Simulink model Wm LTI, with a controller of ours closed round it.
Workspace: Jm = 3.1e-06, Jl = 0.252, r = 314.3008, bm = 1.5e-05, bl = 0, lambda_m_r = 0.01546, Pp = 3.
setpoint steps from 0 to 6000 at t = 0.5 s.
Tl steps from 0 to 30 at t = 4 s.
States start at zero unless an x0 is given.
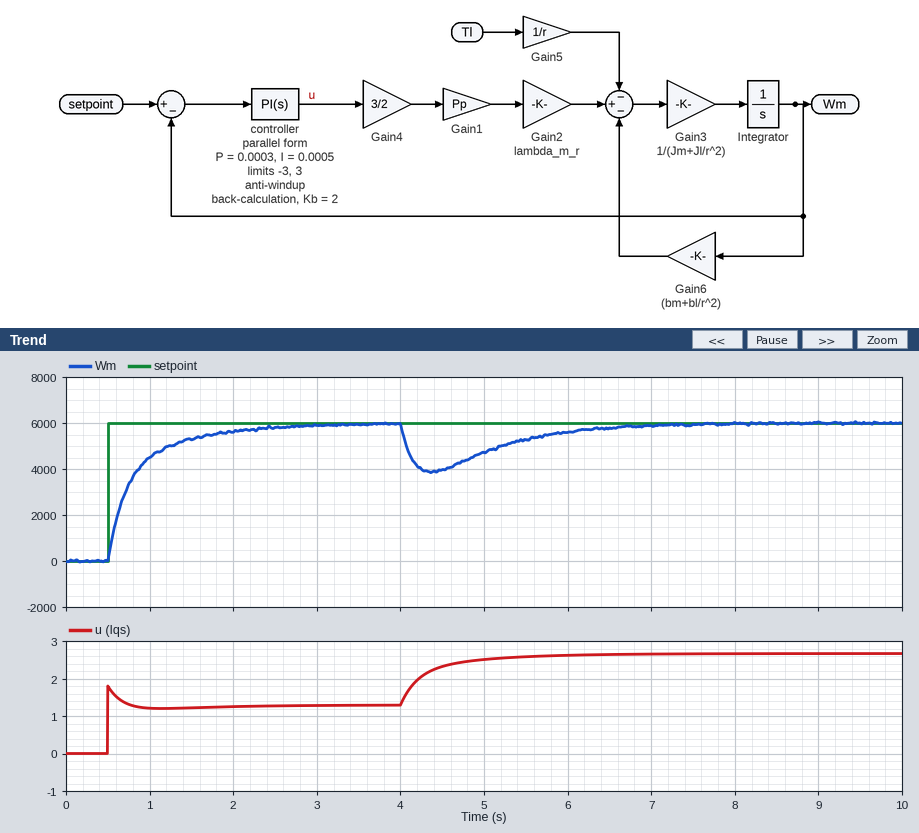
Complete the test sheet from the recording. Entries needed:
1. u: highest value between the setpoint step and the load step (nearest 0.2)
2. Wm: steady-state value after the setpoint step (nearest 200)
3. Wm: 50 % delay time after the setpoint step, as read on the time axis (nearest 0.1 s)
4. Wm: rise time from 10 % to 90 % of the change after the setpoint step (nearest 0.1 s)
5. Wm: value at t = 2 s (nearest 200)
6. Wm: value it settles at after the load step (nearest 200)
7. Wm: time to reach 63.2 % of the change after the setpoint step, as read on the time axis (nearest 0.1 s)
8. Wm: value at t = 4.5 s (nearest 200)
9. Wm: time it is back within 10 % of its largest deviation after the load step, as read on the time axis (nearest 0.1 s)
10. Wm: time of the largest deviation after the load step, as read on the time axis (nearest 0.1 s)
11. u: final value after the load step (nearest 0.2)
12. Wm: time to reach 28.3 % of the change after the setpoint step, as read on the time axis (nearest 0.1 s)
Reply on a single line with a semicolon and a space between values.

1.8; 6000; 0.7 s; 1.1 s; 5600; 6000; 0.8 s; 4000; 6.5 s; 4.4 s; 2.6; 0.6 s
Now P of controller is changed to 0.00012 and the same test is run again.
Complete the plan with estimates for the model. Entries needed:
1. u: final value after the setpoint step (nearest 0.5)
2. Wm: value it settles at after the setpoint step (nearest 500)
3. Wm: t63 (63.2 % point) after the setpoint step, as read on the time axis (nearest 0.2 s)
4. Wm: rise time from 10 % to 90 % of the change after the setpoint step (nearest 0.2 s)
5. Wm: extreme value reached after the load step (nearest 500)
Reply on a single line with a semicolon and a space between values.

1.5; 6000; 1.0 s; 0.8 s; 3000
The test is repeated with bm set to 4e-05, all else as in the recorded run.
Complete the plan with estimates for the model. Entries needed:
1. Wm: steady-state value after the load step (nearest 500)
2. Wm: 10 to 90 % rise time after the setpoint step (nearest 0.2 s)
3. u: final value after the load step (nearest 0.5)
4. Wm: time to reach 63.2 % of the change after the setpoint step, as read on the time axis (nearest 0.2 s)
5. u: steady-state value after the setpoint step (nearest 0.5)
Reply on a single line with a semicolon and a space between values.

3000; 1.8 s; 3.0; 1.2 s; 3.0
